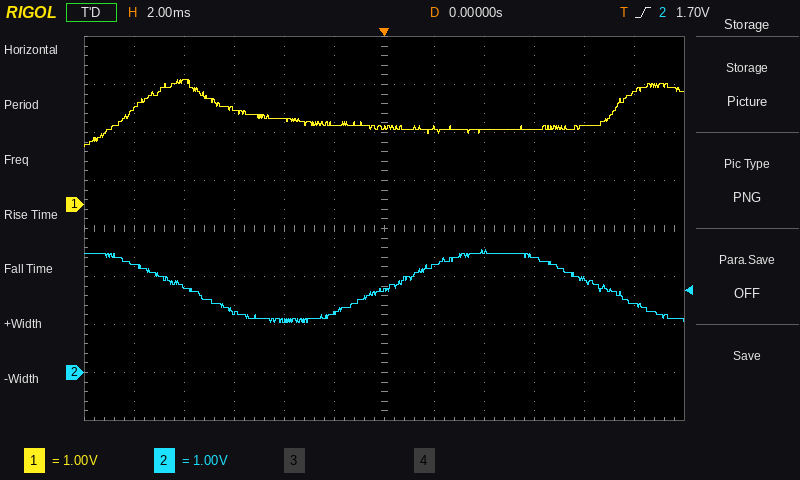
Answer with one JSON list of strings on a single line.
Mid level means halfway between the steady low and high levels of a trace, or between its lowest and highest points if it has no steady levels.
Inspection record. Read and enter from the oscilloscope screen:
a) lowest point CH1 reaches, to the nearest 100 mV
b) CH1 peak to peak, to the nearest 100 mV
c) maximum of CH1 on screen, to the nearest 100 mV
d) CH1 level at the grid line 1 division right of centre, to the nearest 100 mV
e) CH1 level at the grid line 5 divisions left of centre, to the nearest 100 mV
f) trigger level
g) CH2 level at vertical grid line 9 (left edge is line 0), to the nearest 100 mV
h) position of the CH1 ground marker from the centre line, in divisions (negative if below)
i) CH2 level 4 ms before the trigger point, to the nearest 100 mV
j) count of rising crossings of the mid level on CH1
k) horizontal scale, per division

["1.2 V", "1.4 V", "2.6 V", "1.6 V", "2.0 V", "1.70 V", "2.4 V", "+0.5 div", "1.1 V", "2", "2 ms"]
